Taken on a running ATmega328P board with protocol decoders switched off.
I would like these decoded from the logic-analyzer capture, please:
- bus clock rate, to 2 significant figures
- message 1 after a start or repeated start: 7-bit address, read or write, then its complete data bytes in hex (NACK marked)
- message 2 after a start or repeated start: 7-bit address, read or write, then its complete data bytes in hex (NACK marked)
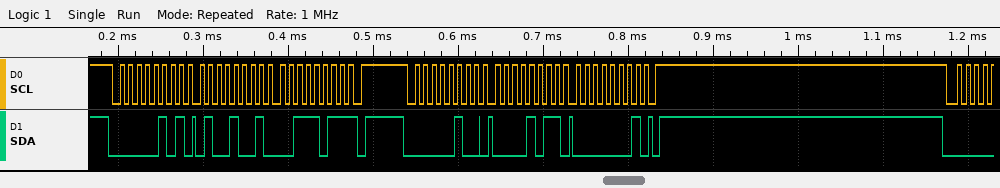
100 kHz
0x02 read: 49 3B NACK
0x02 write: 0B 01
